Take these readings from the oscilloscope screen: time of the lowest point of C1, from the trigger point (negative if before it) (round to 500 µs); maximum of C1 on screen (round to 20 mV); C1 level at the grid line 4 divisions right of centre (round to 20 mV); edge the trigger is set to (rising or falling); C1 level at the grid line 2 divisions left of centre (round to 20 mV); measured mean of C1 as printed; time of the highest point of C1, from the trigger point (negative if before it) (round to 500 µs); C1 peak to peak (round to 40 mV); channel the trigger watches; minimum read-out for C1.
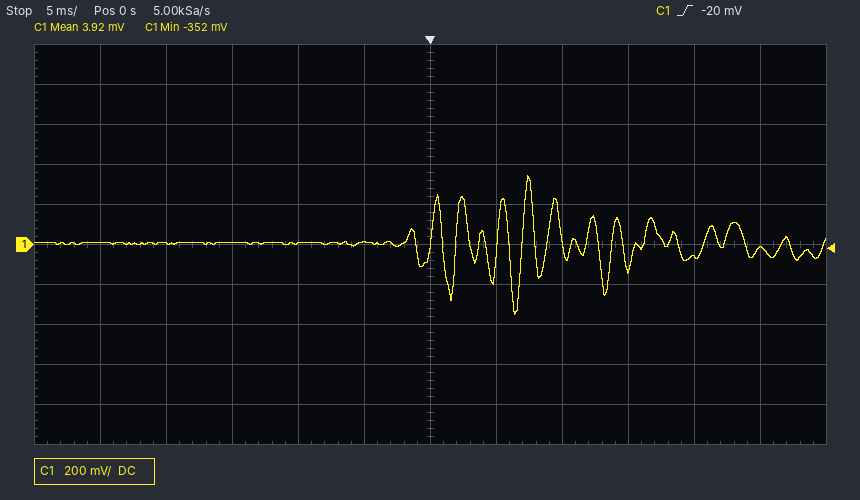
+6.5 ms
340 mV
-60 mV
rising
0 mV
3.92 mV
+7.5 ms
680 mV
C1
-352 mV
